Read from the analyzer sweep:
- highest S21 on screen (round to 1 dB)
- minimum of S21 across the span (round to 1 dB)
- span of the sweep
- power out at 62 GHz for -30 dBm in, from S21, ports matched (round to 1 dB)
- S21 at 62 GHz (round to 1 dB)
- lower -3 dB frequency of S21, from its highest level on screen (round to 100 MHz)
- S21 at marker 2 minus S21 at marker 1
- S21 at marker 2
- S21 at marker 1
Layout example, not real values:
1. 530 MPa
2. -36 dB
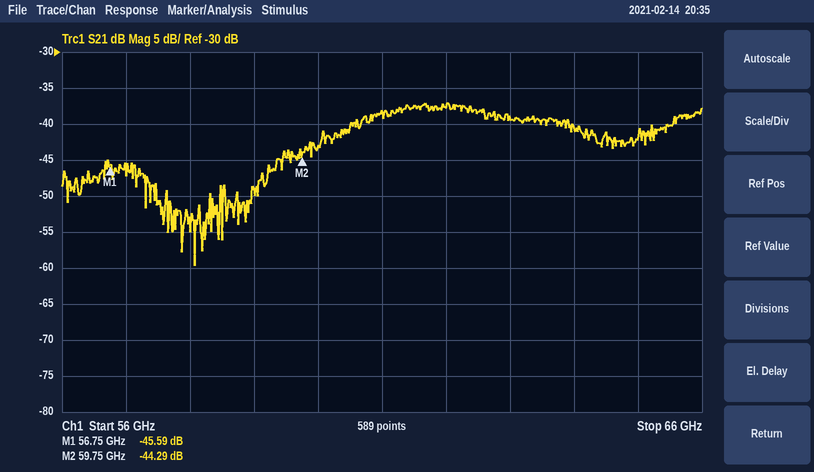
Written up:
1. -37 dB
2. -60 dB
3. 10 GHz
4. -68 dBm
5. -38 dB
6. 60.7 GHz
7. 1.30 dB
8. -44.29 dB
9. -45.59 dB
